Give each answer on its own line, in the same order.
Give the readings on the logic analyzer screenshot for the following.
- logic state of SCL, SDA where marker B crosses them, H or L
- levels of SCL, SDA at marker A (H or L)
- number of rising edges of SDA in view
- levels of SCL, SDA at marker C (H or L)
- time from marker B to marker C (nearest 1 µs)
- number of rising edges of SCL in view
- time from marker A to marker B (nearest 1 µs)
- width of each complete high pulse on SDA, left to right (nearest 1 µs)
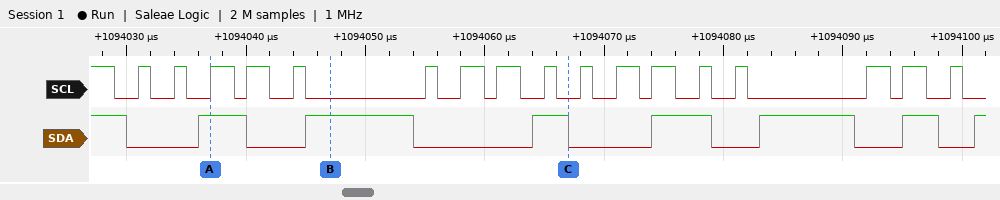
SCL=L, SDA=H
SCL=H, SDA=H
7
SCL=L, SDA=L
20 µs
17
10 µs
4 µs, 9 µs, 3 µs, 5 µs, 8 µs, 3 µs
